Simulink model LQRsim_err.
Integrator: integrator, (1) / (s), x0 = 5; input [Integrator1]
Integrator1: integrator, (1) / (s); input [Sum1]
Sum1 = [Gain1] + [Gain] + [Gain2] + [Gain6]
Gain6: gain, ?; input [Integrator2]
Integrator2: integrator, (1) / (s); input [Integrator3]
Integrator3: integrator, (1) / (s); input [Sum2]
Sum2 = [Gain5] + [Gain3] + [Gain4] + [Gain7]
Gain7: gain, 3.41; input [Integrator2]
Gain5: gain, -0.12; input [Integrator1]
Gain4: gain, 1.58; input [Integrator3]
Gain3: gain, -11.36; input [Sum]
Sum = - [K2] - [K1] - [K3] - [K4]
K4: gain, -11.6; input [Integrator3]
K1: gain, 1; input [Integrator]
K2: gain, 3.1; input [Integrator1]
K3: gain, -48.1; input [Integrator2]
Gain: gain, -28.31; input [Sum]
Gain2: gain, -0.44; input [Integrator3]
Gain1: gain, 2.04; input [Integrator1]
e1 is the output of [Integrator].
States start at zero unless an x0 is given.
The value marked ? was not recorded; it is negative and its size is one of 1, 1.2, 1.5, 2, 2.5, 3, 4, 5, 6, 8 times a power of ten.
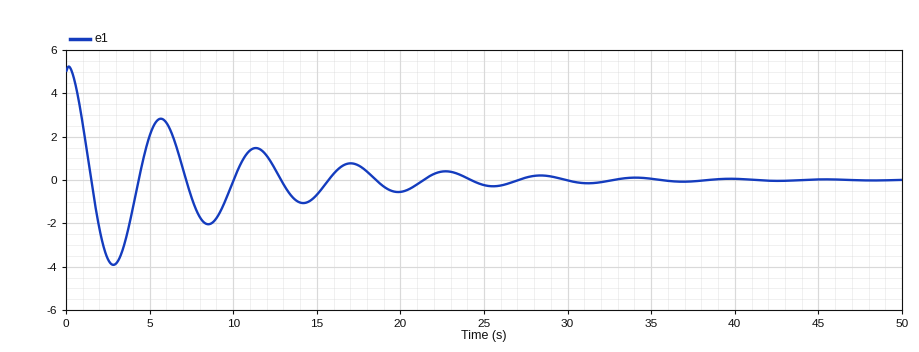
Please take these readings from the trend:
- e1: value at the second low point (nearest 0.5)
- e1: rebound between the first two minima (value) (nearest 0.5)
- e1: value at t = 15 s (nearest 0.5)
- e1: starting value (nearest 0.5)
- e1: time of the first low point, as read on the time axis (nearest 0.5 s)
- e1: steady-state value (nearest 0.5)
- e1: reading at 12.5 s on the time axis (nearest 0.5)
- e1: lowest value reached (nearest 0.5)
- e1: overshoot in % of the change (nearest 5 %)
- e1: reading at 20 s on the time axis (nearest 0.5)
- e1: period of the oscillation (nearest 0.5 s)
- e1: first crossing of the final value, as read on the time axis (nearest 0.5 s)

-2.0
3.0
-0.5
5.0
3.0 s
0.0
0.5
-4.0
80 %
-0.5
5.5 s
1.5 s
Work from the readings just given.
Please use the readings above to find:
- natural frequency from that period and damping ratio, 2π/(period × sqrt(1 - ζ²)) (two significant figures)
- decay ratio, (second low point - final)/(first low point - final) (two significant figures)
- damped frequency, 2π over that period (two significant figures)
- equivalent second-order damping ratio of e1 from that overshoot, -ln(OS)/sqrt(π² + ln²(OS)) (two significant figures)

1.1 rad/s
0.50
1.1 rad/s
0.071
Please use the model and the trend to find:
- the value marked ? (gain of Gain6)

-30
